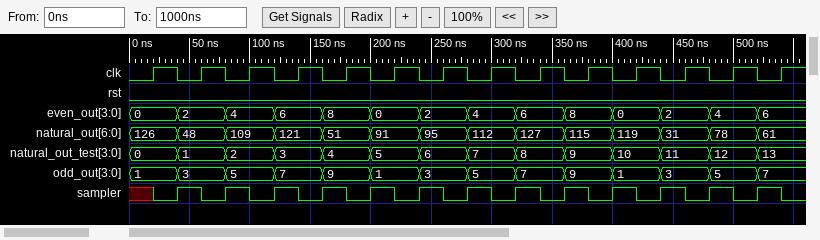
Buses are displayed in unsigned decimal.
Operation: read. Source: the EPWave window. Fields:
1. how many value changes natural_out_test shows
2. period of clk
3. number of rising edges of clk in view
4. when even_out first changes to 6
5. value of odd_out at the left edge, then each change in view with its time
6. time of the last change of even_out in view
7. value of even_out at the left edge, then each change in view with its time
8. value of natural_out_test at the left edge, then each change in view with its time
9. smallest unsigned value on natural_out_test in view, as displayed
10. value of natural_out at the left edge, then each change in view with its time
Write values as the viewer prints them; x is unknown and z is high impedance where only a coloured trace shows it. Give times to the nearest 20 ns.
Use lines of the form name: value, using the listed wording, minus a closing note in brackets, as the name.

how many value changes natural_out_test shows: 13
period of clk: 40 ns
number of rising edges of clk in view: 14
when even_out first changes to 6: 120 ns
value of odd_out at the left edge, then each change in view with its time: 1, 3 at 40 ns, 5 at 80 ns, 7 at 120 ns, 9 at 160 ns, 1 at 200 ns, 3 at 240 ns, 5 at 280 ns, 7 at 320 ns, 9 at 360 ns, 1 at 400 ns, 3 at 440 ns, 5 at 480 ns, 7 at 520 ns
time of the last change of even_out in view: 520 ns
value of even_out at the left edge, then each change in view with its time: 0, 2 at 40 ns, 4 at 80 ns, 6 at 120 ns, 8 at 160 ns, 0 at 200 ns, 2 at 240 ns, 4 at 280 ns, 6 at 320 ns, 8 at 360 ns, 0 at 400 ns, 2 at 440 ns, 4 at 480 ns, 6 at 520 ns
value of natural_out_test at the left edge, then each change in view with its time: 0, 1 at 40 ns, 2 at 80 ns, 3 at 120 ns, 4 at 160 ns, 5 at 200 ns, 6 at 240 ns, 7 at 280 ns, 8 at 320 ns, 9 at 360 ns, 10 at 400 ns, 11 at 440 ns, 12 at 480 ns, 13 at 520 ns
smallest unsigned value on natural_out_test in view, as displayed: 0
value of natural_out at the left edge, then each change in view with its time: 126, 48 at 40 ns, 109 at 80 ns, 121 at 120 ns, 51 at 160 ns, 91 at 200 ns, 95 at 240 ns, 112 at 280 ns, 127 at 320 ns, 115 at 360 ns, 119 at 400 ns, 31 at 440 ns, 78 at 480 ns, 61 at 520 ns
